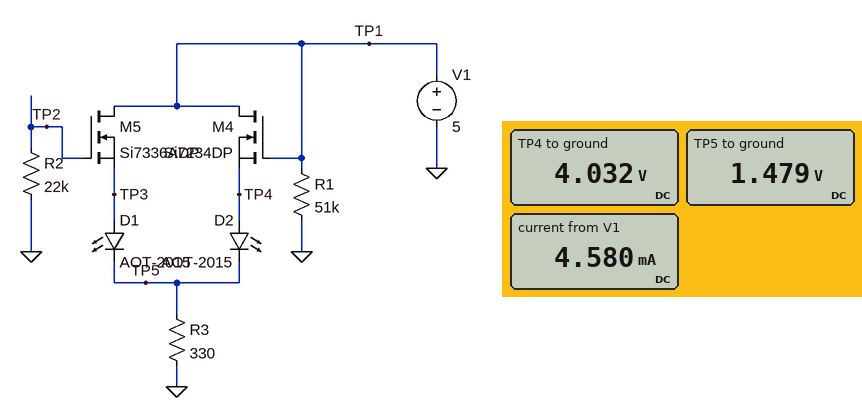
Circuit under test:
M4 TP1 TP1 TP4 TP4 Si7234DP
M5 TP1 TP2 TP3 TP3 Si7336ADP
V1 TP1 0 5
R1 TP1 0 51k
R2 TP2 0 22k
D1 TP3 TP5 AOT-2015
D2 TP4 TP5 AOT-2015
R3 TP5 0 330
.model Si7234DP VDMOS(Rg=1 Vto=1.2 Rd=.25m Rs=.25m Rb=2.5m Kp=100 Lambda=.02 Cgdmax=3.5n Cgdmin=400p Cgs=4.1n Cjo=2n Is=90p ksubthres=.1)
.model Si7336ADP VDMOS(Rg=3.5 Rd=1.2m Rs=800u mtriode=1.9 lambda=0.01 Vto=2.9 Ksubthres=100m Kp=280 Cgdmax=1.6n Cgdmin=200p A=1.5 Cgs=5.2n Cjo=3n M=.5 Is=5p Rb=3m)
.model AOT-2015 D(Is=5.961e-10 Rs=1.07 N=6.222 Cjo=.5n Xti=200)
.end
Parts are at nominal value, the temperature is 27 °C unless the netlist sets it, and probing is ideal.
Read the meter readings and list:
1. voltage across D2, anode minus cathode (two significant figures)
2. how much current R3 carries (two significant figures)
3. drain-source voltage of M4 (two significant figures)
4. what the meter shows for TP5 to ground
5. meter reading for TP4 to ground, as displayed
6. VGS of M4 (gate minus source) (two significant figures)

2.6 V
4.5 mA
970 mV
1.479 V
4.032 V
970 mV
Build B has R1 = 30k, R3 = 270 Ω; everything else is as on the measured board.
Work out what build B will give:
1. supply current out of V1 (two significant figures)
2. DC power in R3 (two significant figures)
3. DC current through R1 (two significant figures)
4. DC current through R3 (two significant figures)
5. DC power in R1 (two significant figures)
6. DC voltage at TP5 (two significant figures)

5.5 mA
7.7 mW
170 µA
5.3 mA
830 µW
1.4 V
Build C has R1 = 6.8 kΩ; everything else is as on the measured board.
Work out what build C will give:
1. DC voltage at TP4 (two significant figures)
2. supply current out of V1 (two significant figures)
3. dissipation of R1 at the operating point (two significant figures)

4.0 V
5.2 mA
3.7 mW
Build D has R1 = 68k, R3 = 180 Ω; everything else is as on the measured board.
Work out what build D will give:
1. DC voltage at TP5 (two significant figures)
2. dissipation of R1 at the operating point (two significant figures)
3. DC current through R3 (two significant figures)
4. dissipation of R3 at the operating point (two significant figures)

1.4 V
370 µW
7.6 mA
10 mW
